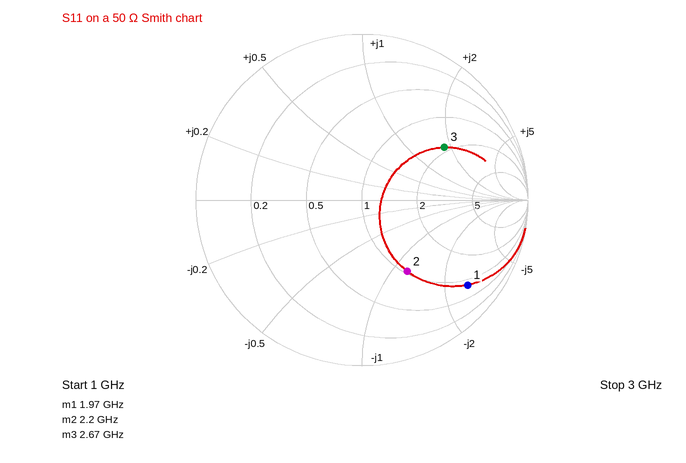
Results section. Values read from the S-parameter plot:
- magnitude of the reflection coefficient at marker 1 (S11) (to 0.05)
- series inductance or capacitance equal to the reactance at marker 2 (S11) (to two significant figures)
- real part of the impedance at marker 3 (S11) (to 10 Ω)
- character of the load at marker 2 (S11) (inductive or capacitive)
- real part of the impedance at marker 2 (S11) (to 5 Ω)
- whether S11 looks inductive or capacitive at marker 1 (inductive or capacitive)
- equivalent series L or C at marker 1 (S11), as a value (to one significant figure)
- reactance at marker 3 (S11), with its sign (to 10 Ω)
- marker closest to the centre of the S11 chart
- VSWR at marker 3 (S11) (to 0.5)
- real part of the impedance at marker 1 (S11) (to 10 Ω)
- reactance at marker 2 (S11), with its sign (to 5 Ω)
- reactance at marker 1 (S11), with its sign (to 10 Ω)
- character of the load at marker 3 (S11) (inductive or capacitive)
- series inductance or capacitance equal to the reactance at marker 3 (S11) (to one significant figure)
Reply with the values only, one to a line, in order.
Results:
0.80
1.2 pF
90 Ω
capacitive
50 Ω
capacitive
600 fF
+90 Ω
marker 2
4.0
40 Ω
-60 Ω
-130 Ω
inductive
5 nH
